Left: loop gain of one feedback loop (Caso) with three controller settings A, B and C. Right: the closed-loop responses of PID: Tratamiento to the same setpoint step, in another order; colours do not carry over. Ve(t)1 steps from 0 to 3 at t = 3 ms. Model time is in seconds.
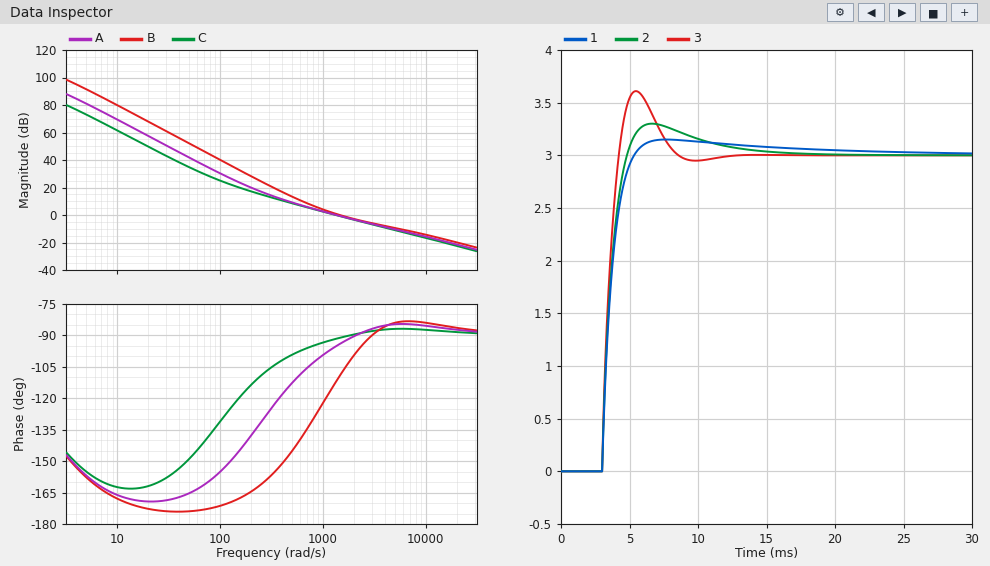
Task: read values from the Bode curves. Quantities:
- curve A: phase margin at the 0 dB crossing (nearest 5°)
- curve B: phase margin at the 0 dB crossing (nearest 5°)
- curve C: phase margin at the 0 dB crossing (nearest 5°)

85°
70°
90°
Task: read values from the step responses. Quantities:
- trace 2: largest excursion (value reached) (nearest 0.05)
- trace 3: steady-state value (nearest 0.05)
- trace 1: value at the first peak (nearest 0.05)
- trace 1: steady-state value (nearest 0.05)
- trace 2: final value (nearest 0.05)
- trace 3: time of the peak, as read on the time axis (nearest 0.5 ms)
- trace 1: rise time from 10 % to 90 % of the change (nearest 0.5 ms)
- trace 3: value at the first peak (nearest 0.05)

3.30
3.00
3.15
3.00
3.00
5.5 ms
1.5 ms
3.60
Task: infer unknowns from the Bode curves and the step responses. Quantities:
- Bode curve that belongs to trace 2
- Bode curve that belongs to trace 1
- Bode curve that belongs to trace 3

A
C
B
